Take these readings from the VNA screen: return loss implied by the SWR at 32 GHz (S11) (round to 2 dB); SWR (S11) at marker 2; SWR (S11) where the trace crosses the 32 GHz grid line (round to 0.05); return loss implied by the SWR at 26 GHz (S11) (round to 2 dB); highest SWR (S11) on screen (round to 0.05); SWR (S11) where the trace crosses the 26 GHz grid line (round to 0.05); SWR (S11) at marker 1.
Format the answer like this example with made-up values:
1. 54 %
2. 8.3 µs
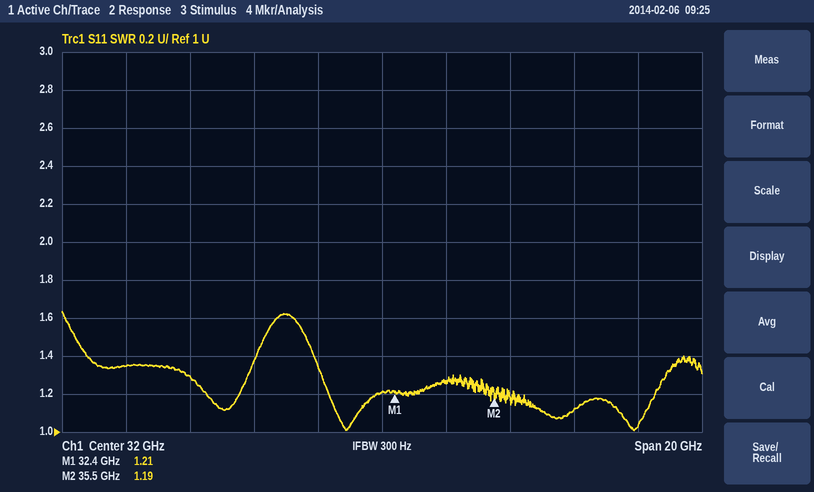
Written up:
1. 20 dB
2. 1.19
3. 1.20
4. 18 dB
5. 1.65
6. 1.30
7. 1.21
